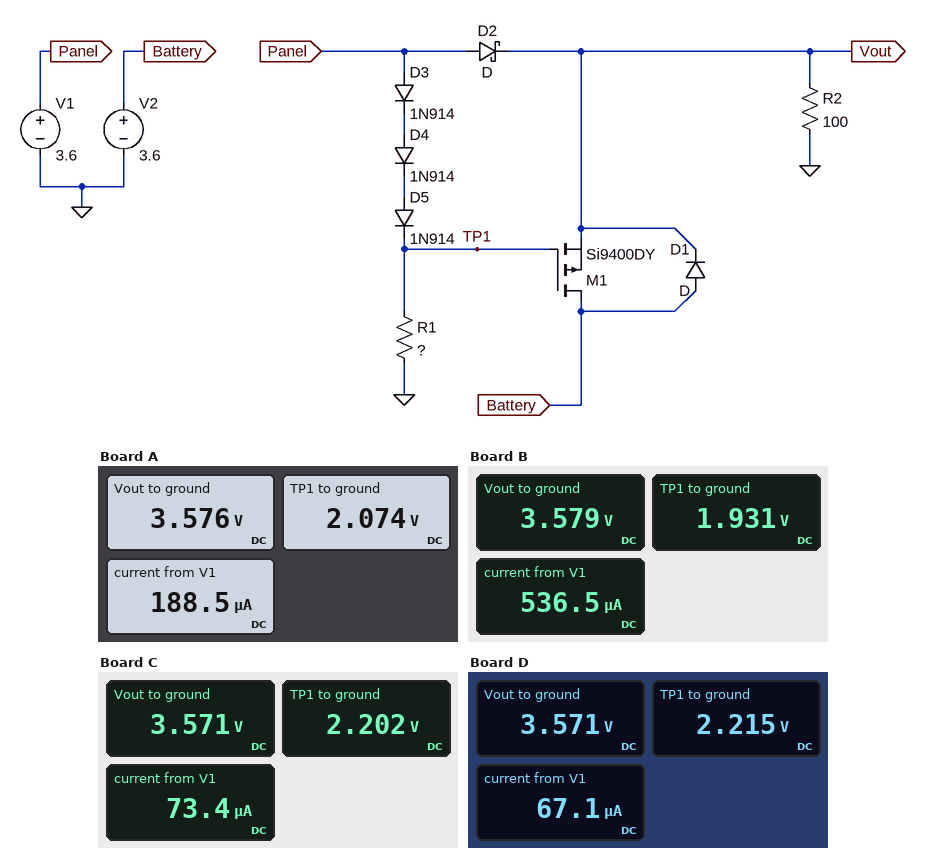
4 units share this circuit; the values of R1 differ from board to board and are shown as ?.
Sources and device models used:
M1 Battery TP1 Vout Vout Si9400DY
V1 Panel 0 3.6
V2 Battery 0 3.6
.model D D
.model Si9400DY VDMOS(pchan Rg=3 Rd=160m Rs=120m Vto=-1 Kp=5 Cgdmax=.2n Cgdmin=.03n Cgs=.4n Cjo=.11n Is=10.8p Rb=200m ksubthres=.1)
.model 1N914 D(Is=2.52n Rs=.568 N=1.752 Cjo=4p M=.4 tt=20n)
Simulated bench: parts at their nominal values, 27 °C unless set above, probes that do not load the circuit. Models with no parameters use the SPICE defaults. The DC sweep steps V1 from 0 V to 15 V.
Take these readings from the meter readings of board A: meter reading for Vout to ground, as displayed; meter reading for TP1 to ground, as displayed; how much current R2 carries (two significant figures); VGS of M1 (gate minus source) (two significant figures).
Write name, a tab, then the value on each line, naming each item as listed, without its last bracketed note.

meter reading for Vout to ground, as displayed	3.576 V
meter reading for TP1 to ground, as displayed	2.074 V
how much current R2 carries	36 mA
VGS of M1 (gate minus source)	-1.5 V
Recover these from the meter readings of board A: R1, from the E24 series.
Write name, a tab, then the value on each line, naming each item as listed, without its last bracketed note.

R1, from the E24 series	11 kΩ
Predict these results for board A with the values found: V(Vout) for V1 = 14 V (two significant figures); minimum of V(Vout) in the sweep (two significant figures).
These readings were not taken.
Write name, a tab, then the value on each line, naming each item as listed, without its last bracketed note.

V(Vout) for V1 = 14 V	13 V
minimum of V(Vout) in the sweep	3.4 V
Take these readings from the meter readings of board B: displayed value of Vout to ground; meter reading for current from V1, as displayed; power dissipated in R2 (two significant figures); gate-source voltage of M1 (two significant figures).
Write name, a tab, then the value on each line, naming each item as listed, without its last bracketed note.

displayed value of Vout to ground	3.579 V
meter reading for current from V1, as displayed	536.5 µA
power dissipated in R2	130 mW
gate-source voltage of M1	-1.6 V
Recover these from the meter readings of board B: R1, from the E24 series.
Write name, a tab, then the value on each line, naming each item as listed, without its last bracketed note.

R1, from the E24 series	3.6 kΩ
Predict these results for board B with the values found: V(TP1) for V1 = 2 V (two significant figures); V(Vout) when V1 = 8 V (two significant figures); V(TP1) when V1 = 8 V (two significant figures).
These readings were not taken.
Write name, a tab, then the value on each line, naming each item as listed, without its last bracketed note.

V(TP1) for V1 = 2 V	510 mV
V(Vout) when V1 = 8 V	7.2 V
V(TP1) when V1 = 8 V	6.2 V
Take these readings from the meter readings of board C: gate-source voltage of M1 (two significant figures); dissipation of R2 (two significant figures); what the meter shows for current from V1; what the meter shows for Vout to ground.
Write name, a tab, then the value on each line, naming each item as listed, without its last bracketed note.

gate-source voltage of M1	-1.4 V
dissipation of R2	130 mW
what the meter shows for current from V1	73.4 µA
what the meter shows for Vout to ground	3.571 V
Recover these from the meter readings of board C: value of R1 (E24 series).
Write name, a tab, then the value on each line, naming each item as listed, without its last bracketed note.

value of R1	30 kΩ
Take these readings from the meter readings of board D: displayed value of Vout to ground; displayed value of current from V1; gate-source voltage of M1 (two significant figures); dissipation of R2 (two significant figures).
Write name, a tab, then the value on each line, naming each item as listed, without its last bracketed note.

displayed value of Vout to ground	3.571 V
displayed value of current from V1	67.1 µA
gate-source voltage of M1	-1.4 V
dissipation of R2	130 mW
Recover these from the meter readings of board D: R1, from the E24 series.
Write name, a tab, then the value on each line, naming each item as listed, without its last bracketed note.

R1, from the E24 series	33 kΩ
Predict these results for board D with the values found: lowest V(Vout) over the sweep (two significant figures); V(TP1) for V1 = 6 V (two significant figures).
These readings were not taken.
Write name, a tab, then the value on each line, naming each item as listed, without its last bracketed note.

lowest V(Vout) over the sweep	3.2 V
V(TP1) for V1 = 6 V	4.5 V
